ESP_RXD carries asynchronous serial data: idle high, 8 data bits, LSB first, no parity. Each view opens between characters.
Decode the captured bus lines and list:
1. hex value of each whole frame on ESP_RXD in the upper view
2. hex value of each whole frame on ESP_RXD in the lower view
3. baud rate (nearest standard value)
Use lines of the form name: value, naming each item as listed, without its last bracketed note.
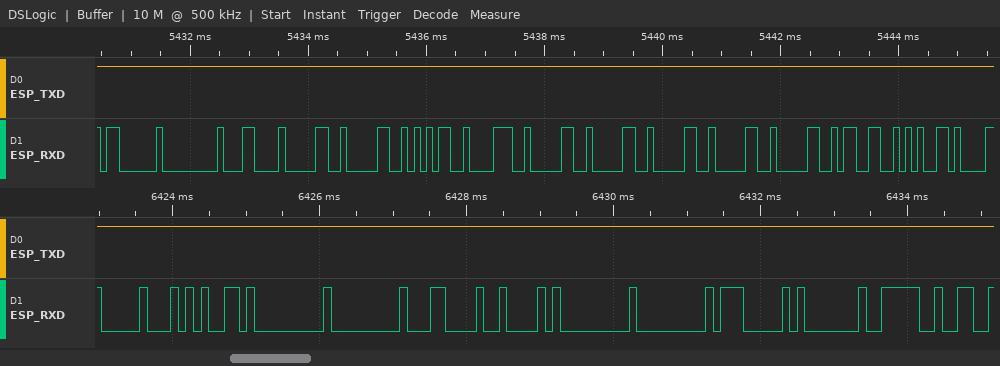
hex value of each whole frame on ESP_RXD in the upper view: 03, 00, 0C, 30, 30, 35, 38, 30, 30, 30, 30, 30, 33, 65
hex value of each whole frame on ESP_RXD in the lower view: 10, 65, 00, 00, 0C, 42, 00, 00, 07, 01, 3E
baud rate: 9600 baud
